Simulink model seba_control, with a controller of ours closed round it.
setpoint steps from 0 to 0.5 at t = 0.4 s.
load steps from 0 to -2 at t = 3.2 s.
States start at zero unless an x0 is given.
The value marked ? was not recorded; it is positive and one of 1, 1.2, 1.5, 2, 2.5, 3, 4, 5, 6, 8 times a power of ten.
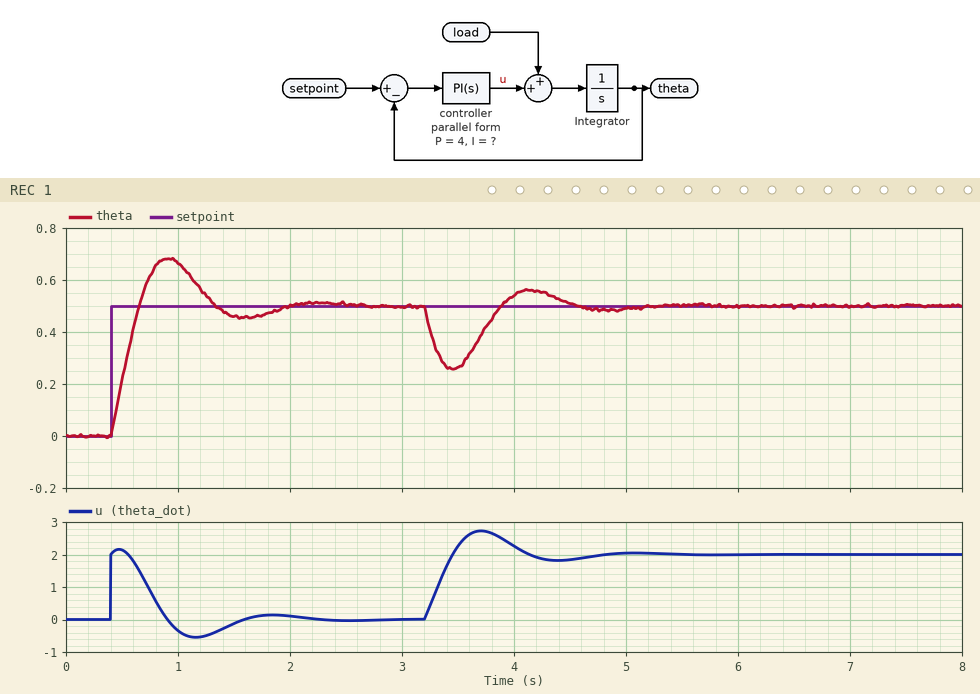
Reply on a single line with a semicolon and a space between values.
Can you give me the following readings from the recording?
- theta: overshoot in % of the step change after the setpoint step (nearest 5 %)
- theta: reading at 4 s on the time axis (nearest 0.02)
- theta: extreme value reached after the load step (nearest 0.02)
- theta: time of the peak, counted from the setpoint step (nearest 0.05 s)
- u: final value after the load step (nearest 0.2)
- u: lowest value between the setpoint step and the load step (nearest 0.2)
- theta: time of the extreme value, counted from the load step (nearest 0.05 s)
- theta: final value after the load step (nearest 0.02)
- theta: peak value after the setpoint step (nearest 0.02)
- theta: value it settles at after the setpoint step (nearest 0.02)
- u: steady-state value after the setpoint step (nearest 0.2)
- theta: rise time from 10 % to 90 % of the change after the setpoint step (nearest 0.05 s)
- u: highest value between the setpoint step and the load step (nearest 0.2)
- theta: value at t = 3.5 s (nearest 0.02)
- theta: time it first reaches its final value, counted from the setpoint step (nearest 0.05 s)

35 %; 0.54; 0.26; 0.50 s; 2.0; -0.6; 0.25 s; 0.50; 0.68; 0.50; 0.0; 0.20 s; 2.2; 0.26; 0.25 s
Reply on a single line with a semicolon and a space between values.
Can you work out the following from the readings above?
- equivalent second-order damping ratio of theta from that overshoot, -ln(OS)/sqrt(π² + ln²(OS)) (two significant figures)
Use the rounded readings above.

0.32
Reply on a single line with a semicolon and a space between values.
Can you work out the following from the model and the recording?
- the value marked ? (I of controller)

25
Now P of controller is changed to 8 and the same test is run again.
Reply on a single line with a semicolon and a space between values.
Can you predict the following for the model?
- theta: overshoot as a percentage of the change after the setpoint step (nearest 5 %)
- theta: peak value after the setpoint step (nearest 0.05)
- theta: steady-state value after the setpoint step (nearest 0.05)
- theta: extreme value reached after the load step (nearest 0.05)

20 %; 0.60; 0.50; 0.35
